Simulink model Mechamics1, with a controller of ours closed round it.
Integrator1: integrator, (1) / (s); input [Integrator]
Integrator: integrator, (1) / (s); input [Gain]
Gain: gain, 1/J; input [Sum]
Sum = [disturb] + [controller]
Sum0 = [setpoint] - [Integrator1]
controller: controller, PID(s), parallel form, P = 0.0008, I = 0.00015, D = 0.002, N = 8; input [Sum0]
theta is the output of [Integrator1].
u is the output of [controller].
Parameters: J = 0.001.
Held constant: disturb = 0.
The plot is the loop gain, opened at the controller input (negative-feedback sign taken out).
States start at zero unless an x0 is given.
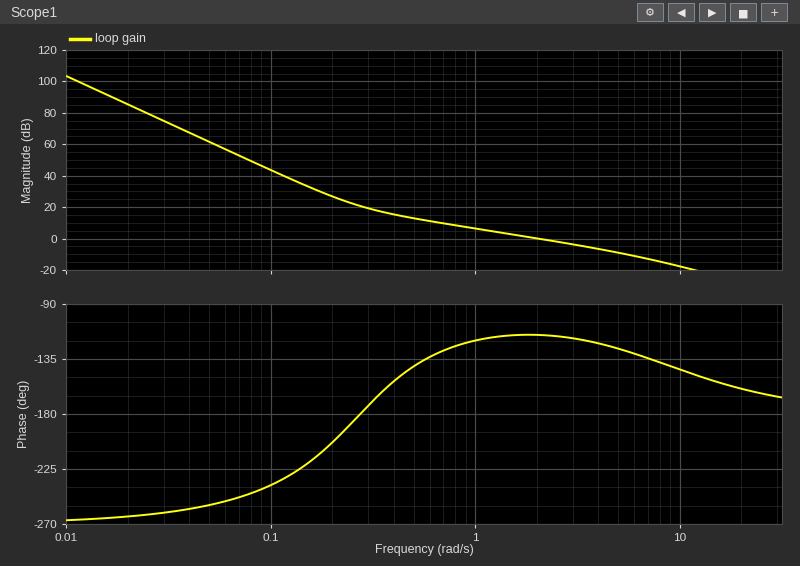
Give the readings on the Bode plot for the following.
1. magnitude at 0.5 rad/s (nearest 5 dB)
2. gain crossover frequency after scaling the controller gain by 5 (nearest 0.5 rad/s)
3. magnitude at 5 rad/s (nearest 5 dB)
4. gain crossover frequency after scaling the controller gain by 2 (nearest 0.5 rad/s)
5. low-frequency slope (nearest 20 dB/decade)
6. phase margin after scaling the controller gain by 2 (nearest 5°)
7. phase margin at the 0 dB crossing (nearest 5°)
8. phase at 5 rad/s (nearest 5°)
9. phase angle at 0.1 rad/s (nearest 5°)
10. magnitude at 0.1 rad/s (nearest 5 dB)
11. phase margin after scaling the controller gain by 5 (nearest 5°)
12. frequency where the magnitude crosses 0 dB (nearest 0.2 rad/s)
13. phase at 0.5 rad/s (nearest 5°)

15 dB
7.5 rad/s
-10 dB
4.0 rad/s
-60 dB/decade
60°
65°
-125°
-240°
45 dB
45°
2.0 rad/s
-140°
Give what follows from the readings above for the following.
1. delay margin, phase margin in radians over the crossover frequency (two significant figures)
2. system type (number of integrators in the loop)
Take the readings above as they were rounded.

0.57 s
3
